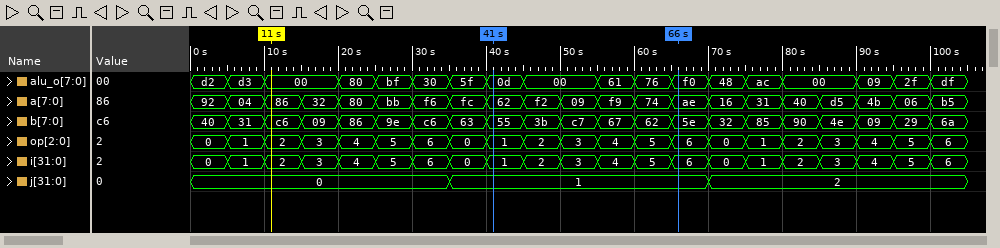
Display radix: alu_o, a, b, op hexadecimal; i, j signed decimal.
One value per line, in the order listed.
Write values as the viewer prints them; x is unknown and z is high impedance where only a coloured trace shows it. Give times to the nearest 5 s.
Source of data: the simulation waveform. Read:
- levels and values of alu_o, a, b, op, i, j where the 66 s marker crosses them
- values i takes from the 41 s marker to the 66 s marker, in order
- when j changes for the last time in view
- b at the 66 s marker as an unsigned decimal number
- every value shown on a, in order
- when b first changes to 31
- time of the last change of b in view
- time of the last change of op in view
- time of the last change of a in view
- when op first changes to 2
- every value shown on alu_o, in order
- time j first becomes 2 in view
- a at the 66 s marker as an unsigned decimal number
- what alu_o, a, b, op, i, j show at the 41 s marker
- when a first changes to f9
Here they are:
alu_o=f0, a=ae, b=5e, op=6, i=6, j=1
1, 2, 3, 4, 5, 6
70 s
94
92, 04, 86, 32, 80, bb, f6, fc, 62, f2, 09, f9, 74, ae, 16, 31, 40, d5, 4b, 06, b5
5 s
100 s
100 s
100 s
10 s
d2, d3, 00, 80, bf, 30, 5f, 0d, 00, 61, 76, f0, 48, ac, 00, 09, 2f, df
70 s
174
alu_o=0d, a=62, b=55, op=1, i=1, j=1
55 s
